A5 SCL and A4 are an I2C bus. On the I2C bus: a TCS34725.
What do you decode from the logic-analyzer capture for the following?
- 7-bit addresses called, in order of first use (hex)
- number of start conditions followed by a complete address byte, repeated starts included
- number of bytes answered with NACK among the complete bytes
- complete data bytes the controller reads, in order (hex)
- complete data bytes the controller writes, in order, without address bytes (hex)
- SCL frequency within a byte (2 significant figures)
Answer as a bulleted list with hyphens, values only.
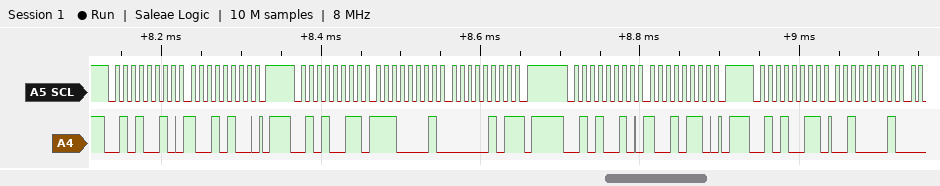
- 0x29
- 4
- 1
- E1 05 21
- 94 96
- 100 kHz
